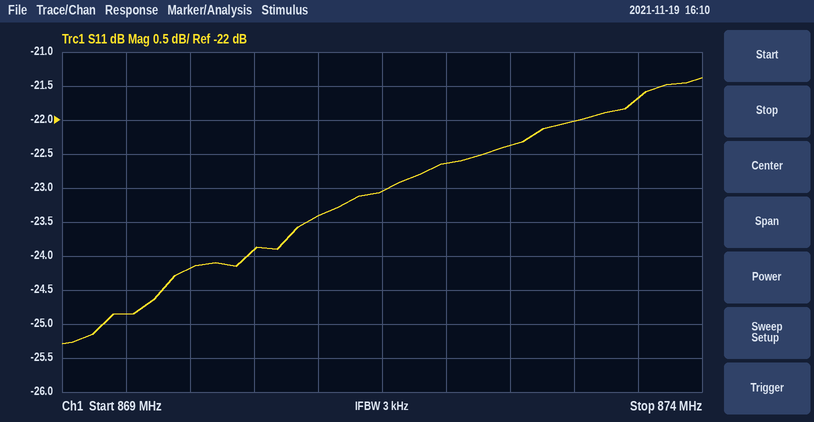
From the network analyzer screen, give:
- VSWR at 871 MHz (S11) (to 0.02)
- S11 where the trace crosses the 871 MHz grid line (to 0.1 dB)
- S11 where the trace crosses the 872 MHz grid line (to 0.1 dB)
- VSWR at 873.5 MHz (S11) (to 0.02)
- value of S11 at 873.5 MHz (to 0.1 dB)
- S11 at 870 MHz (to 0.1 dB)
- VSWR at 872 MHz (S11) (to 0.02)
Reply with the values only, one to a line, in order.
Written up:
1.14
-23.4 dB
-22.6 dB
1.18
-21.7 dB
-24.2 dB
1.16
